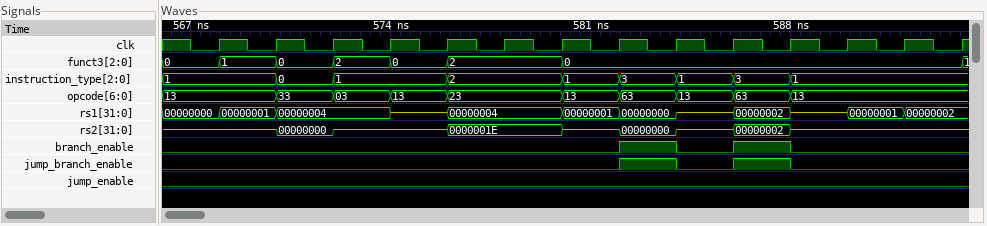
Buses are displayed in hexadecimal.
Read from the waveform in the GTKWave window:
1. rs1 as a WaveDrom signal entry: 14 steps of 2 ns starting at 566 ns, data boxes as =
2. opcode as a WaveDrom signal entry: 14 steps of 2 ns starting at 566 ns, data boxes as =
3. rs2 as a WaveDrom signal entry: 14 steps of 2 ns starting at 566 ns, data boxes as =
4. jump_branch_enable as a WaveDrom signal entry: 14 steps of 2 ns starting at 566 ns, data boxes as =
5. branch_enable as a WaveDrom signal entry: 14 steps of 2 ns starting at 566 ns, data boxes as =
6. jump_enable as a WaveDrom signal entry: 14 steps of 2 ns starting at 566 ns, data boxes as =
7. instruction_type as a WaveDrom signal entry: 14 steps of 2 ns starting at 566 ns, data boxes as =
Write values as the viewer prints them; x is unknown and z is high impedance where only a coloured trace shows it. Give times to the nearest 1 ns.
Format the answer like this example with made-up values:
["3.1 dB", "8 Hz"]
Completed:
["{name: 'rs1', wave: '===.z=.==z=z==', data: '00000000 00000001 00000004 00000004 00000001 00000000 00000002 00000001 00000002'}", "{name: 'opcode', wave: '=.====.=====..', data: '13 33 03 13 23 13 63 13 63 13'}", "{name: 'rs2', wave: 'z.=z.=.z=z=z..', data: '00000000 0000001E 00000000 00000002'}", "{name: 'jump_branch_enable', wave: '0.......1010..'}", "{name: 'branch_enable', wave: '0.......1010..'}", "{name: 'jump_enable', wave: '0.............'}", "{name: 'instruction_type', wave: '=.==.=.=====..', data: '1 0 1 2 1 3 1 3 1'}"]
